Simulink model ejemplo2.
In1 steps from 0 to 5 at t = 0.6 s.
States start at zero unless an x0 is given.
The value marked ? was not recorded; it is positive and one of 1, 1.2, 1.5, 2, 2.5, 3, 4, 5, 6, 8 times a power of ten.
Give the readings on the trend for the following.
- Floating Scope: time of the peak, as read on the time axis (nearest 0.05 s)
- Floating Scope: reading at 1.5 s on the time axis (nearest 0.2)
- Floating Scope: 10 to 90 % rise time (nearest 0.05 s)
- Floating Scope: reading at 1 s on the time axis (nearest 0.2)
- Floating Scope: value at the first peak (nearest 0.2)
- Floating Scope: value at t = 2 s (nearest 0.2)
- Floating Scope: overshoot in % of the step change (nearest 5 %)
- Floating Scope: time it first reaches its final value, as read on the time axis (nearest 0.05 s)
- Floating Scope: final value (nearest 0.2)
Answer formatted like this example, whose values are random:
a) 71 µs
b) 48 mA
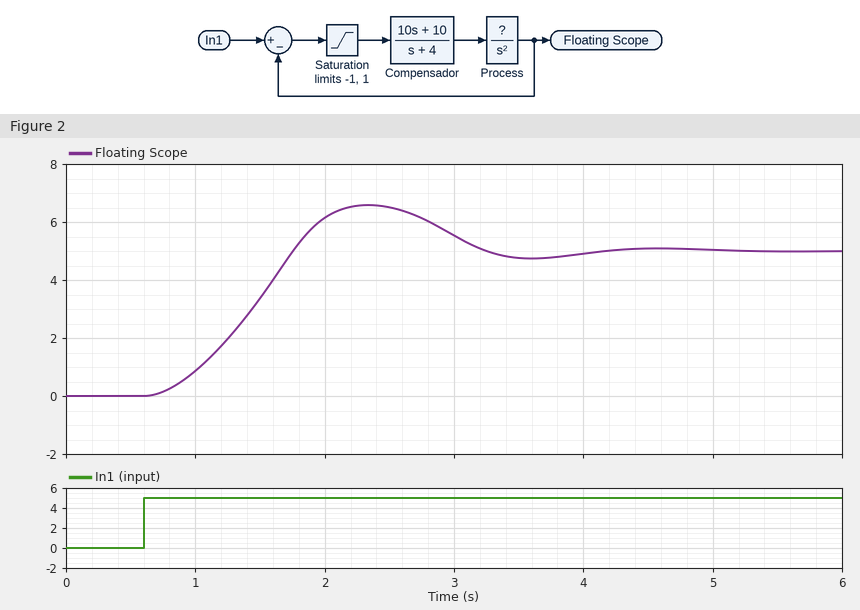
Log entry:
a) 2.35 s
b) 3.4
c) 0.80 s
d) 0.8
e) 6.6
f) 6.2
g) 30 %
h) 1.75 s
i) 5.0
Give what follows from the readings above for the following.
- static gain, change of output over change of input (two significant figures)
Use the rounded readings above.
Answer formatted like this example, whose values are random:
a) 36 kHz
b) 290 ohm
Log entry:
a) 1.0
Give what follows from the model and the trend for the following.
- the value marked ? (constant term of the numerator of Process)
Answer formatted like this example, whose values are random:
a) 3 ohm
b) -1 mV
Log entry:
a) 1.5
